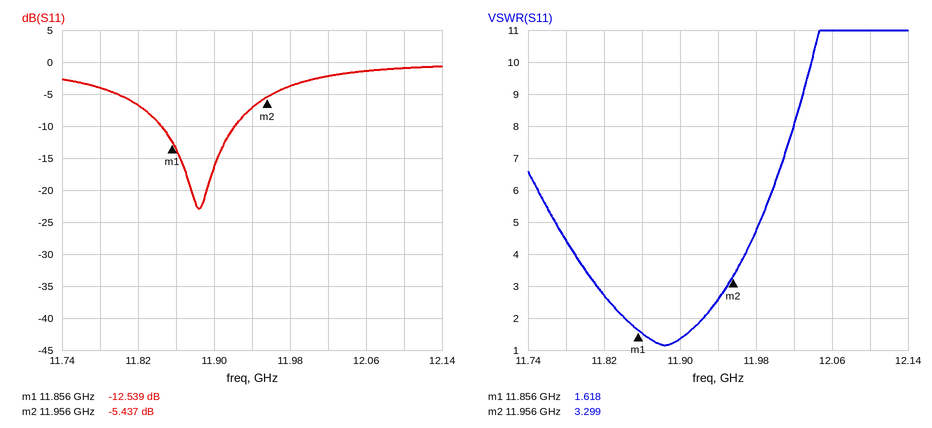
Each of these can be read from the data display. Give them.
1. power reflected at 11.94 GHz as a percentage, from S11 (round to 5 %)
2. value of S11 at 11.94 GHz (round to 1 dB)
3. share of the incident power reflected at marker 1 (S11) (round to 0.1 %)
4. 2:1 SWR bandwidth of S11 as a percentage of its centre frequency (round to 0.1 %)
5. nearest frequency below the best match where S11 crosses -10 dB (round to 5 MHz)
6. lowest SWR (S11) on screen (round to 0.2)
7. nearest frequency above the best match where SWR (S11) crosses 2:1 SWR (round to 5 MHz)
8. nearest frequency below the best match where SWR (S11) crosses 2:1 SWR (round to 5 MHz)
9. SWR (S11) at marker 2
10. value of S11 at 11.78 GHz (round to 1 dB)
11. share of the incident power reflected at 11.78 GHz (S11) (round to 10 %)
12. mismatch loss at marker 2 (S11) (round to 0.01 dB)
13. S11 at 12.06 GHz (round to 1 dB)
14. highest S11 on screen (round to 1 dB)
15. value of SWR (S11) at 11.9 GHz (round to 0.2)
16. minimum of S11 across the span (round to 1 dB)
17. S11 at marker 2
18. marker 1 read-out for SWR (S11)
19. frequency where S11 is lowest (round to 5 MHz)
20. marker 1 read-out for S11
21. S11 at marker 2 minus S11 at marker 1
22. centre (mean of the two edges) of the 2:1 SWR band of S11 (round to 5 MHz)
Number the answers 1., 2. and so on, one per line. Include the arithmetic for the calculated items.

1. 10^(-7/10) ≈ 20 %
2. -7 dB
3. 10^(-12.539/10) ≈ 5.6 %
4. 85 MHz / 11.8825 GHz ≈ 0.7 %
5. 11.845 GHz
6. 1.2
7. 11.925 GHz
8. 11.840 GHz
9. 3.299
10. -4 dB
11. 10^(-4/10) ≈ 40 %
12. −10 log10(1 − 10^(-5.437/10)) ≈ 1.46 dB
13. -1 dB
14. -1 dB
15. 1.4
16. -23 dB
17. -5.437 dB
18. 1.618
19. 11.885 GHz
20. -12.539 dB
21. -5.437 − (-12.539) = 7.102 dB
22. 11.885 GHz
